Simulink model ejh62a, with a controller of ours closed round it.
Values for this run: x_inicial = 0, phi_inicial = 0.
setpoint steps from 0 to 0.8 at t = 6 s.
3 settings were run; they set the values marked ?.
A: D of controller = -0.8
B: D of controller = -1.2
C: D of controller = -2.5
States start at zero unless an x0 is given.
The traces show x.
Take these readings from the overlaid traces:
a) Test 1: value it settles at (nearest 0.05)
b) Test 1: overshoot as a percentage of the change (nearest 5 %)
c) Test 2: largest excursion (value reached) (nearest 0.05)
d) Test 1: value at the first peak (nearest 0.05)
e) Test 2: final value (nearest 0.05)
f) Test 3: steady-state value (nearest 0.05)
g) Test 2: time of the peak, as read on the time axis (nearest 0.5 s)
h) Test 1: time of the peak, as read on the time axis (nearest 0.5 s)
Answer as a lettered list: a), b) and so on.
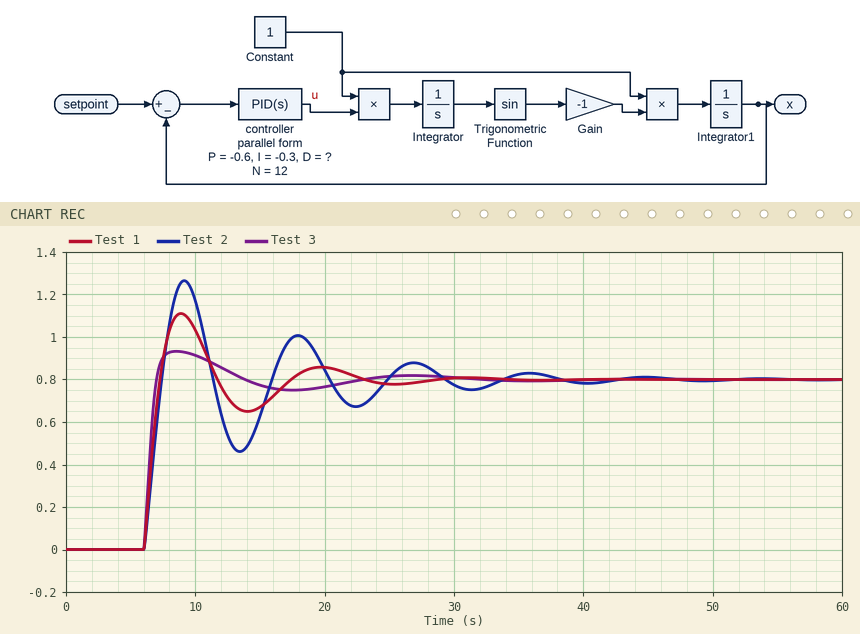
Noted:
a) 0.80
b) 40 %
c) 1.25
d) 1.10
e) 0.80
f) 0.80
g) 9.0 s
h) 9.0 s
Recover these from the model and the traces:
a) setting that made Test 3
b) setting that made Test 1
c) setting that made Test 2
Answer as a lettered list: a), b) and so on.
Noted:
a) C
b) B
c) A
